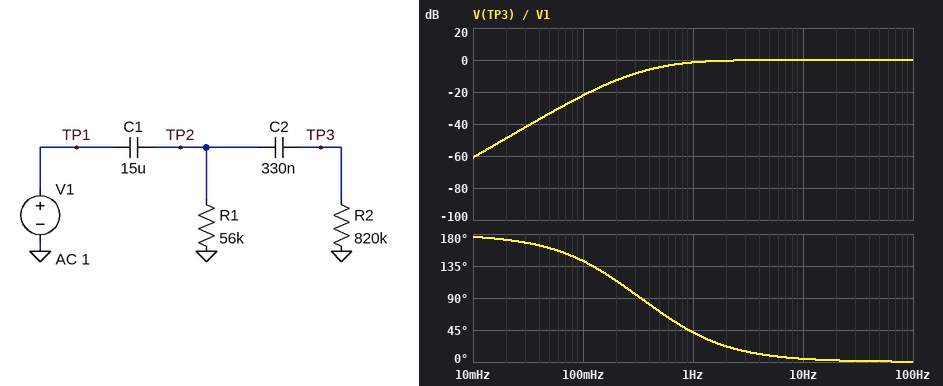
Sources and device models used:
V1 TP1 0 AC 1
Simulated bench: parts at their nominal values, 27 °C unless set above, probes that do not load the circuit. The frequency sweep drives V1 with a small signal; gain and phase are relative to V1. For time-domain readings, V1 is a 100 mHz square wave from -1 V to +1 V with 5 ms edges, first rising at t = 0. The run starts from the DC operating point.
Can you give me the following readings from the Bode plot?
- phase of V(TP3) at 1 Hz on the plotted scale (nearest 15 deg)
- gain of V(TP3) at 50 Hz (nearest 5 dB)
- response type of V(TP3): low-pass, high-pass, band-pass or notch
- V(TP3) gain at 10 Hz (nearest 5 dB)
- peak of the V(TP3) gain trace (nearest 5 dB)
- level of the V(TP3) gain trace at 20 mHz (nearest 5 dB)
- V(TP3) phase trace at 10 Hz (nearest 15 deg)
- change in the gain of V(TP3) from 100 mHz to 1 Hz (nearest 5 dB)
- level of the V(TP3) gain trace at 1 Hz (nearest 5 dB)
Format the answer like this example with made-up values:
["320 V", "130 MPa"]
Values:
["45 deg", "0 dB", "high-pass", "0 dB", "0 dB", "-50 dB", "0 deg", "20 dB", "0 dB"]
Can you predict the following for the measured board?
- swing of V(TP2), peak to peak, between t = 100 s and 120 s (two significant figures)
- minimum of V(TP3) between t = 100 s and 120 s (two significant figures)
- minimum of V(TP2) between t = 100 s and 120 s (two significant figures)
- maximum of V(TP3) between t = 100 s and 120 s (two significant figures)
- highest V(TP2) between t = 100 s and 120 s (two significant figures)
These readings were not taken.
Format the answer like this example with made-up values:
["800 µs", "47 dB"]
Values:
["4.0 V", "-2.0 V", "-2.0 V", "2.0 V", "2.0 V"]
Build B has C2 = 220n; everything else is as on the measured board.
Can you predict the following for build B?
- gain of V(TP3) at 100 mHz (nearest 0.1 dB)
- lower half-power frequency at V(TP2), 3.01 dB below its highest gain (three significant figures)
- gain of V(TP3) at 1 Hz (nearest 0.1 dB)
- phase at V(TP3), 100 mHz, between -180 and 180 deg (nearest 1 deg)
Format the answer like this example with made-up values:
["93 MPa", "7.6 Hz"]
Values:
["-25.6 dB", "193 mHz", "-2.7 dB", "145 deg"]
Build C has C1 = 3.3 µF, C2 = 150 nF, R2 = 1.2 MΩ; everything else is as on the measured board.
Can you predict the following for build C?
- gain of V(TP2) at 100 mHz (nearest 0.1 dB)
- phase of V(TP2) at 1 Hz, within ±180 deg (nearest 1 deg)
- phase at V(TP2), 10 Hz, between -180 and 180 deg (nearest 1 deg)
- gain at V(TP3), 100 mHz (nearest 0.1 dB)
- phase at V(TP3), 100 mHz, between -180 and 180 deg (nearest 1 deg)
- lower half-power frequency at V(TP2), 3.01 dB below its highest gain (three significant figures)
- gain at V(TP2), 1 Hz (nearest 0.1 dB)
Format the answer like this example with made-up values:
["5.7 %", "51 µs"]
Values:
["-18.8 dB", "41 deg", "5 deg", "-37.8 dB", "167 deg", "902 mHz", "-2.6 dB"]
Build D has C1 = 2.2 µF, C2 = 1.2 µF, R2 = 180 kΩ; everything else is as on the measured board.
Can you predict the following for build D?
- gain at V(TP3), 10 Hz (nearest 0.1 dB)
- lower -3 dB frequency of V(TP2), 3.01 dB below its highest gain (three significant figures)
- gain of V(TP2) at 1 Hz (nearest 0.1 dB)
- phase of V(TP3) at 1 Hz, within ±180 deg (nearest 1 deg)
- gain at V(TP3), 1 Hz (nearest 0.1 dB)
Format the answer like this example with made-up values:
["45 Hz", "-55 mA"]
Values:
["-0.2 dB", "1.79 Hz", "-5.8 dB", "89 deg", "-7.7 dB"]
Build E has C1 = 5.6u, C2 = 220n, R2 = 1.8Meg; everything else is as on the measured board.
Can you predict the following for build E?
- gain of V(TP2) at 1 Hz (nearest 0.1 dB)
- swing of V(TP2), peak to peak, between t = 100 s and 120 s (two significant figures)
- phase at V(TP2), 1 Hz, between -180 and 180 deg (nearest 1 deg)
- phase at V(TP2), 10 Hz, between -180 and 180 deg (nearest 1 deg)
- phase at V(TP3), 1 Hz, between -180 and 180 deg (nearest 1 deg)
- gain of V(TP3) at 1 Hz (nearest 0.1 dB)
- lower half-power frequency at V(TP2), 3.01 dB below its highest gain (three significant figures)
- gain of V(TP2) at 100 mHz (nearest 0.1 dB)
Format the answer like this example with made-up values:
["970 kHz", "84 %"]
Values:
["-1.1 dB", "4.0 V", "27 deg", "3 deg", "49 deg", "-1.7 dB", "525 mHz", "-14.3 dB"]
